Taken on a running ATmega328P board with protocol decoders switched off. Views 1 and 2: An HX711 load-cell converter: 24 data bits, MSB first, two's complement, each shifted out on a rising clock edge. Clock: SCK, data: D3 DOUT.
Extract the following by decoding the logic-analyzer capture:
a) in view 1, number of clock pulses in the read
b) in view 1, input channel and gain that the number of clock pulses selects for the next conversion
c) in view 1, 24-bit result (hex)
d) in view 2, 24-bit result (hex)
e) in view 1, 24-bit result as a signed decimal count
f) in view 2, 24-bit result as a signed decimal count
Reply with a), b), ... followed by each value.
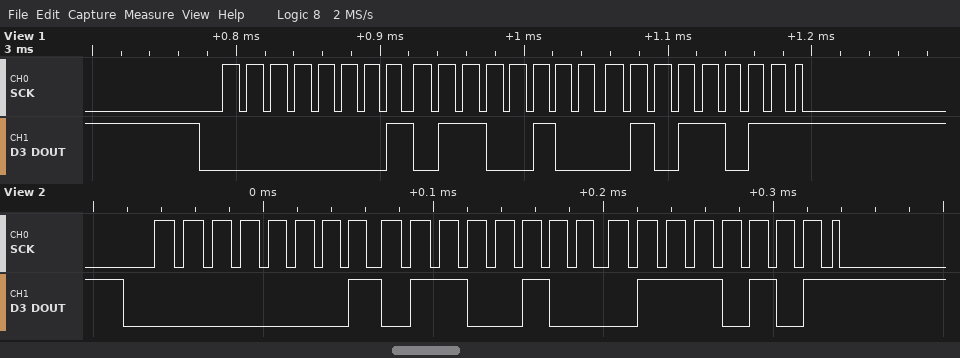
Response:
a) 25
b) channel A, gain 128
c) 0x01645B
d) 0x016475
e) 91227
f) 91253
